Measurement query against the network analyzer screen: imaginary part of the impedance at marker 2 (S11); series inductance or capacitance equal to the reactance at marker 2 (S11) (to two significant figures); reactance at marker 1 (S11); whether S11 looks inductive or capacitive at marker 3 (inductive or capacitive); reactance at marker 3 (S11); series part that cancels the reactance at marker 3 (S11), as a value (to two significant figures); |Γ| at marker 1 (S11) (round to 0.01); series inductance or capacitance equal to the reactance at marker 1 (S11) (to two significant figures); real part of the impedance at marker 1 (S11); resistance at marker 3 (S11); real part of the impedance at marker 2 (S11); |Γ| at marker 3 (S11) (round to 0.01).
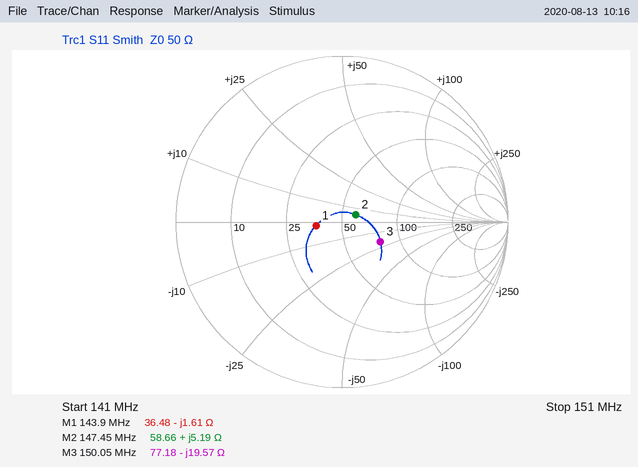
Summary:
+5.19 Ω
5.6 nH
-1.61 Ω
capacitive
-19.57 Ω
21 nH
0.16
690 pF
36.48 Ω
77.18 Ω
58.66 Ω
0.26
